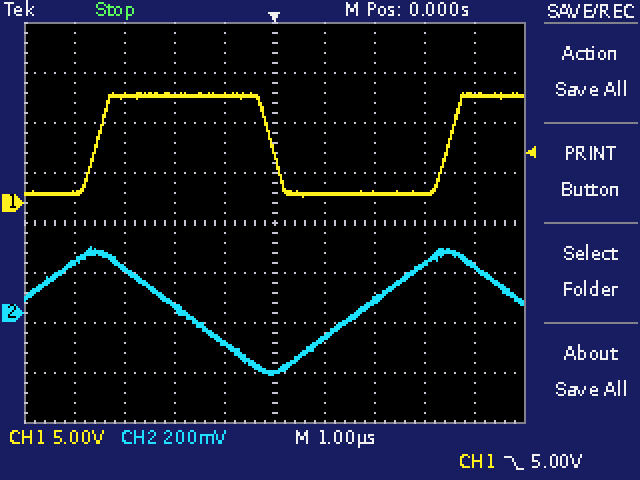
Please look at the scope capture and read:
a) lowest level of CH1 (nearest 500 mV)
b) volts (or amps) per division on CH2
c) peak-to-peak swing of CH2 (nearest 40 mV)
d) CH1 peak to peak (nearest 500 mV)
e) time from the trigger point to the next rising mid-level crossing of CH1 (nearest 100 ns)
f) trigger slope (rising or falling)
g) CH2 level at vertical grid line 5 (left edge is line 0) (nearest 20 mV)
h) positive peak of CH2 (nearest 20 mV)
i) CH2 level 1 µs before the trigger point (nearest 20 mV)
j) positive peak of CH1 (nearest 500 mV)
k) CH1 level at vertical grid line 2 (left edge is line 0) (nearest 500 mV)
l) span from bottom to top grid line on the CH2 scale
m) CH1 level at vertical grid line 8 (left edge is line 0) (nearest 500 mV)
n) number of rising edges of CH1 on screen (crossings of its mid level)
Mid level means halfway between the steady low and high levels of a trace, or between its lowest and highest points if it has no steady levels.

500 mV
200 mV
520 mV
10.5 V
3.5 µs
falling
-240 mV
260 mV
-120 mV
11.0 V
10.5 V
1.6 V
1.0 V
2
